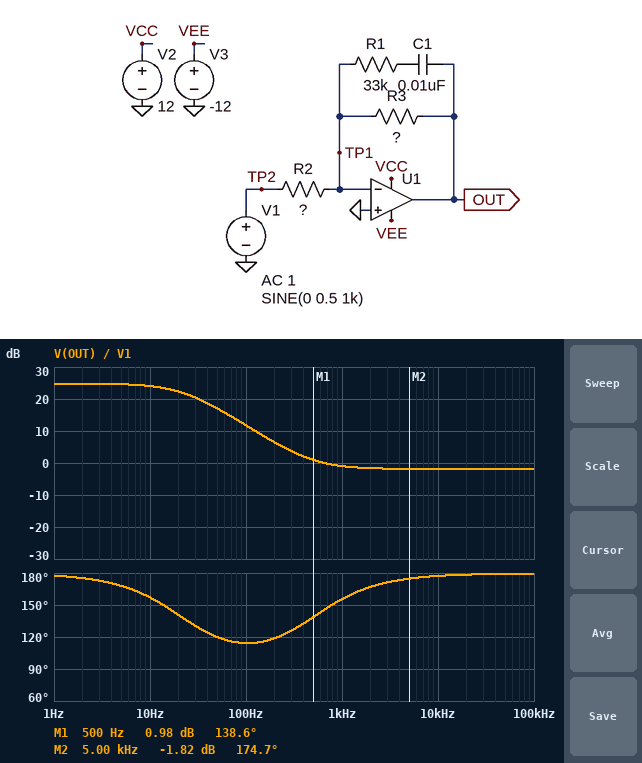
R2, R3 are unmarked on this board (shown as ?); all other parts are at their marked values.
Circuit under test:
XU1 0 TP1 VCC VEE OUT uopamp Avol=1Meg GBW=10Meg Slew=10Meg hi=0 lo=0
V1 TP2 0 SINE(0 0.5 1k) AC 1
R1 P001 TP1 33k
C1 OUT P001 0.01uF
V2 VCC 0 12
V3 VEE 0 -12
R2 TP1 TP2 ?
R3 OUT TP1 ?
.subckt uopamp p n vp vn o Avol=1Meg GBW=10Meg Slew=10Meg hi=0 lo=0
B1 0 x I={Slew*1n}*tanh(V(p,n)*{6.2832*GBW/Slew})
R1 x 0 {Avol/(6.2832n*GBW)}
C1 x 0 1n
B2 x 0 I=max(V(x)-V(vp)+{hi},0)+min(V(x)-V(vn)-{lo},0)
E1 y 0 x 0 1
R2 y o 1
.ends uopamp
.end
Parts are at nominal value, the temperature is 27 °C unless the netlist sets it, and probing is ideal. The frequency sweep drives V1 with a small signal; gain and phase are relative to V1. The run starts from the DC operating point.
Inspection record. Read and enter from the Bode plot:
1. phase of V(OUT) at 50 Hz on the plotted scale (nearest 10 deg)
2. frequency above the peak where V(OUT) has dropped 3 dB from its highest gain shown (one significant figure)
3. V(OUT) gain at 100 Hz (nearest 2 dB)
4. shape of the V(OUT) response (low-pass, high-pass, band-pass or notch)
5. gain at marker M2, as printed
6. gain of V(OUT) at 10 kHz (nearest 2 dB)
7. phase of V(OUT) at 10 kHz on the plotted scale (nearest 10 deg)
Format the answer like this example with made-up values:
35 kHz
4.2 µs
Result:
120 deg
20 Hz
12 dB
low-pass
-1.82 dB
-2 dB
180 deg
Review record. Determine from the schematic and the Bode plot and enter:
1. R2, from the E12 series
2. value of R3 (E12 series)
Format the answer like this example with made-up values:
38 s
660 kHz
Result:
39 kΩ
680 kΩ
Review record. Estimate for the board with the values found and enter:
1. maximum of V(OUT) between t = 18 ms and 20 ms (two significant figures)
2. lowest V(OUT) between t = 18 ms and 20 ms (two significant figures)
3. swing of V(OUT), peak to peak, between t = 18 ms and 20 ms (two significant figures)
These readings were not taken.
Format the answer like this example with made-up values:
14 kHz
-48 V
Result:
440 mV
-460 mV
900 mV
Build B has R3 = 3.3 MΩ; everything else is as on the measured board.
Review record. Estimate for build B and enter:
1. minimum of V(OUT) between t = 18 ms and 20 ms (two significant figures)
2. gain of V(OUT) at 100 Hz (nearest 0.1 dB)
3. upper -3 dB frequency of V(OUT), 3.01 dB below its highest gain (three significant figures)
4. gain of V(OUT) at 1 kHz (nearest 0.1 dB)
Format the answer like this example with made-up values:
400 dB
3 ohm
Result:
-580 mV
12.3 dB
4.78 Hz
-0.6 dB
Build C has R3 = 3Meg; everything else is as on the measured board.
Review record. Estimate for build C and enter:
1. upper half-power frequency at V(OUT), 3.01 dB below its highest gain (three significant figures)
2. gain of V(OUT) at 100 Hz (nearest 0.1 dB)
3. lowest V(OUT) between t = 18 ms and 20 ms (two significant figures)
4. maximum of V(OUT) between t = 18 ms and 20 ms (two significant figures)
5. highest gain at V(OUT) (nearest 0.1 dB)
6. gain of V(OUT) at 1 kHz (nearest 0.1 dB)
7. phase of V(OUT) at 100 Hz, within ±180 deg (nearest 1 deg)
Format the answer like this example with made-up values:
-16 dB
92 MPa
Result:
5.25 Hz
12.3 dB
-570 mV
360 mV
37.7 dB
-0.6 dB
105 deg
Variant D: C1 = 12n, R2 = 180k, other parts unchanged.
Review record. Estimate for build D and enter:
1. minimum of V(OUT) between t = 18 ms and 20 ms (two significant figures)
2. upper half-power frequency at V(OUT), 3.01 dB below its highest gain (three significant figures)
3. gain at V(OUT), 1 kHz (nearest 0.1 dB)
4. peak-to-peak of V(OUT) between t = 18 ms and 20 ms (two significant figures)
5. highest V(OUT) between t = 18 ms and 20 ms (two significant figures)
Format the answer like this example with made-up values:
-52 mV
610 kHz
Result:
-98 mV
18.6 Hz
-14.5 dB
190 mV
91 mV
